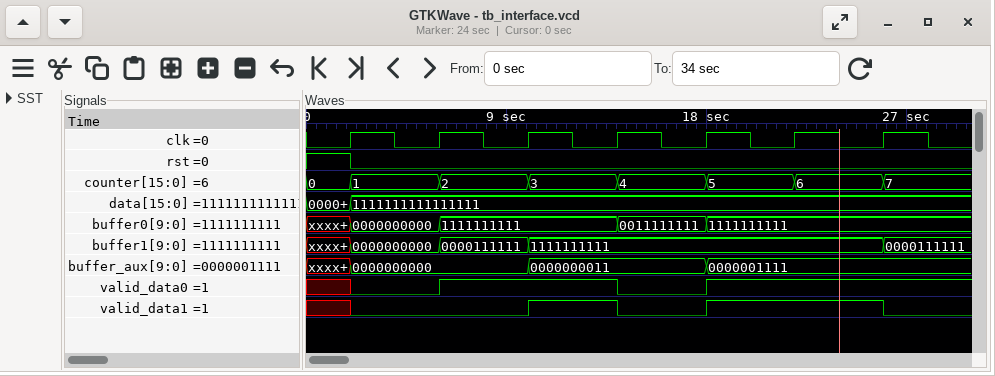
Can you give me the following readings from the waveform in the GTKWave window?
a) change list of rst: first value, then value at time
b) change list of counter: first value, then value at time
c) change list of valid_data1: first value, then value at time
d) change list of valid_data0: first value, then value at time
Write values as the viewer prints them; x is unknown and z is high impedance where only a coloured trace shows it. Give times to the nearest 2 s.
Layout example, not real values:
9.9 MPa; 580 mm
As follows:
1, 0 at 2 s; 0, 1 at 2 s, 2 at 6 s, 3 at 10 s, 4 at 14 s, 5 at 18 s, 6 at 22 s, 7 at 26 s; x, 0 at 2 s, 1 at 10 s, 0 at 14 s, 1 at 18 s, 0 at 26 s; x, 0 at 2 s, 1 at 6 s, 0 at 14 s, 1 at 18 s
